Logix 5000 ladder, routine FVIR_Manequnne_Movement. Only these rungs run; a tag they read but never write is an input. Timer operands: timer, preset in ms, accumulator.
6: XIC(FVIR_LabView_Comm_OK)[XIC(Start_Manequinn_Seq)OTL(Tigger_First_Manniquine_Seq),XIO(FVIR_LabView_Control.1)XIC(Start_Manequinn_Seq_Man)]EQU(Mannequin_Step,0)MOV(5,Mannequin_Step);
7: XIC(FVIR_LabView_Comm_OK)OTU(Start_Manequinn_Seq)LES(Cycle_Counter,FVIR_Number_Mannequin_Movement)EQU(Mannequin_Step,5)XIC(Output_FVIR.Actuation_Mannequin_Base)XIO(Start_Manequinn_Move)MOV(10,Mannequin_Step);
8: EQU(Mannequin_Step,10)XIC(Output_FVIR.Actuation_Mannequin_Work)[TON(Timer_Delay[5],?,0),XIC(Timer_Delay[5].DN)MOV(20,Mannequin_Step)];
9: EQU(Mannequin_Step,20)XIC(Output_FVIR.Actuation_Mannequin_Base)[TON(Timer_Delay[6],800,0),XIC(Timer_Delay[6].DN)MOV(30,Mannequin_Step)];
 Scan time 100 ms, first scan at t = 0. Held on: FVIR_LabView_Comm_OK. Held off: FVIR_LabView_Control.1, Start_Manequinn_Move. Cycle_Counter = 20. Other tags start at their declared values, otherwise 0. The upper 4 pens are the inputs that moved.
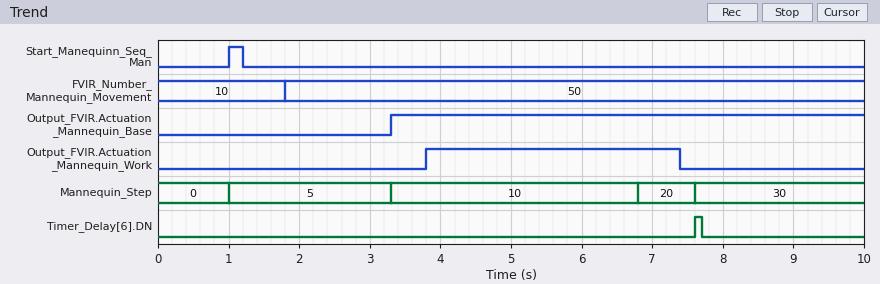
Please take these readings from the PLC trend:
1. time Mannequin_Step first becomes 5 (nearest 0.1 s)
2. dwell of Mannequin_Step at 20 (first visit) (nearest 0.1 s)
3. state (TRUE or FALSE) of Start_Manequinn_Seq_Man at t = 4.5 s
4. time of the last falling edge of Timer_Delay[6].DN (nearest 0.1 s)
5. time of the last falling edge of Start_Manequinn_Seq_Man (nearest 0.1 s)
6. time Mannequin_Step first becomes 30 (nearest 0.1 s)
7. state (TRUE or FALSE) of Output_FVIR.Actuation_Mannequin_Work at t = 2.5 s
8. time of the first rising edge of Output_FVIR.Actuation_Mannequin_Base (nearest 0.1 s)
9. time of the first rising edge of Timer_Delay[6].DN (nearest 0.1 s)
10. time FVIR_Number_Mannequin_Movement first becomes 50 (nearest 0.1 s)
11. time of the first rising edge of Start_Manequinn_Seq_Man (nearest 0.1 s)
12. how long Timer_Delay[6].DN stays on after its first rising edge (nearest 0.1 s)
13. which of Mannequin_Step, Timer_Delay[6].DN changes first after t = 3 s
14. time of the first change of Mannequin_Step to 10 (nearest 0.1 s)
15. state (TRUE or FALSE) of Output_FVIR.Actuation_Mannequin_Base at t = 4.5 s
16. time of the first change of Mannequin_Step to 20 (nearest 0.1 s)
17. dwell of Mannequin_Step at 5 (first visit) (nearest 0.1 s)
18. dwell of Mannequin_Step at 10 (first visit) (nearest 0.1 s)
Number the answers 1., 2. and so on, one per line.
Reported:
1. 1.0 s
2. 0.8 s
3. FALSE
4. 7.7 s
5. 1.2 s
6. 7.6 s
7. FALSE
8. 3.3 s
9. 7.6 s
10. 1.8 s
11. 1.0 s
12. 0.1 s
13. Mannequin_Step
14. 3.3 s
15. TRUE
16. 6.8 s
17. 2.3 s
18. 3.5 s
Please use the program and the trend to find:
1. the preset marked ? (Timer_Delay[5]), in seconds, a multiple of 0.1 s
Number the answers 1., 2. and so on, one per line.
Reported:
1. 3.0 s
